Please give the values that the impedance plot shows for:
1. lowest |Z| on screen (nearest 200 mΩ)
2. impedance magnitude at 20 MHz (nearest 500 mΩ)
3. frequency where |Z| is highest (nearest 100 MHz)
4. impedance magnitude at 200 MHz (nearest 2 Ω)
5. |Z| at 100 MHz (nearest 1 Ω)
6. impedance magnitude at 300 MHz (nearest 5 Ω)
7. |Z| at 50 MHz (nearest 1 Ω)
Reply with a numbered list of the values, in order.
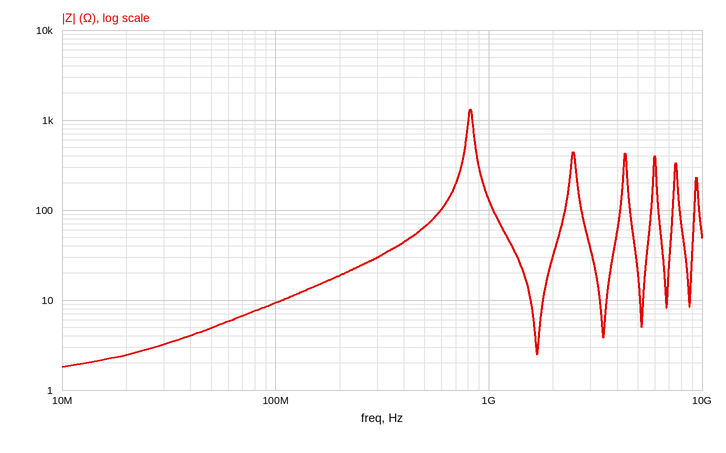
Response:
1. 1.8 Ω
2. 2.5 Ω
3. 800 MHz
4. 18 Ω
5. 9 Ω
6. 30 Ω
7. 5 Ω
